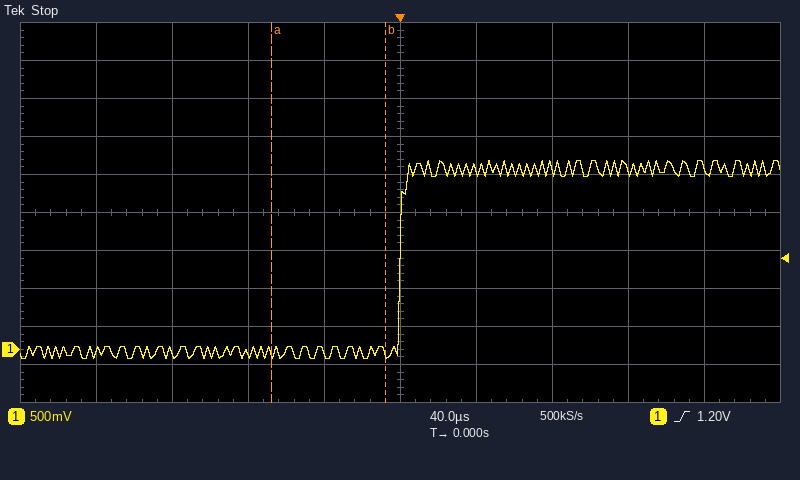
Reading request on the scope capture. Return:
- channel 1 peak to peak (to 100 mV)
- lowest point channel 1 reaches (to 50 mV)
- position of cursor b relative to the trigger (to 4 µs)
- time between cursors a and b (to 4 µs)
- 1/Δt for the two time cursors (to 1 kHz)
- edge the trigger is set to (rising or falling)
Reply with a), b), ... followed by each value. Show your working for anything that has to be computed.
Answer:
a) 2.60 V
b) -100 mV
c) -8 µs
d) 60 µs
e) 1 / 60 µs ≈ 17 kHz
f) rising
